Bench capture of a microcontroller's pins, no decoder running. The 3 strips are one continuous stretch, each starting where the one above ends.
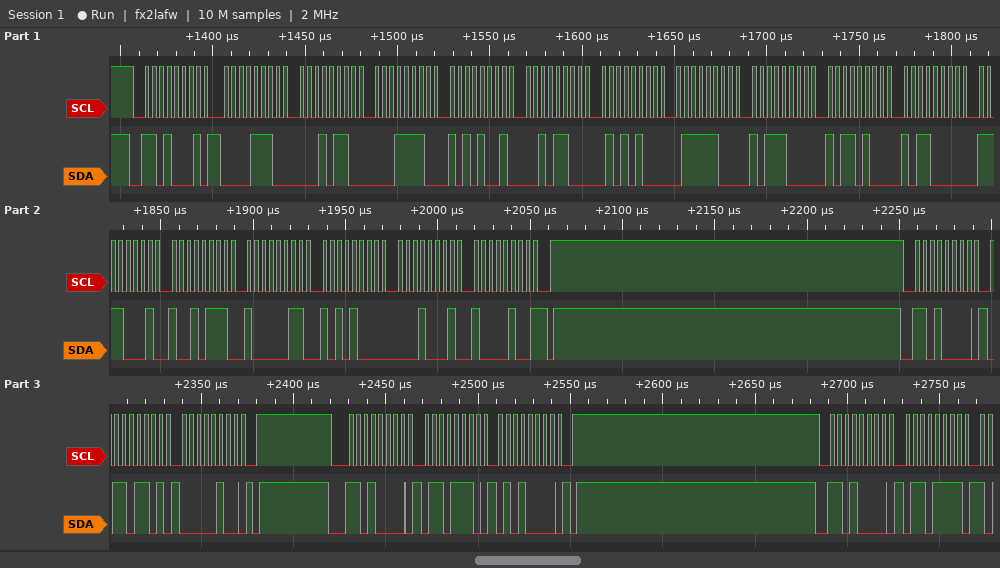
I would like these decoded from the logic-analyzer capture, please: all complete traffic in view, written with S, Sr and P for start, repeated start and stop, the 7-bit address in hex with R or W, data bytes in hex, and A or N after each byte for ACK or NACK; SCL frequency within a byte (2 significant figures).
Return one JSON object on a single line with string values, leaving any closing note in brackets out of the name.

{"all complete traffic in view, written with S, Sr and P for start, repeated start and stop, the 7-bit address in hex with R or W, data bytes in hex, and A or N after each byte for ACK or NACK": "S 68R A 0E A 16 A 1E A A9 A 2C A 54 A 7C A B8 A B4 A B0 A F1 A 97 A 83 A A8 A 11 A 84 N P S 68W A 6D A 04 A P S 68W A 6E A 50 A P S 68W A 6F A", "SCL frequency within a byte": "250 kHz"}
